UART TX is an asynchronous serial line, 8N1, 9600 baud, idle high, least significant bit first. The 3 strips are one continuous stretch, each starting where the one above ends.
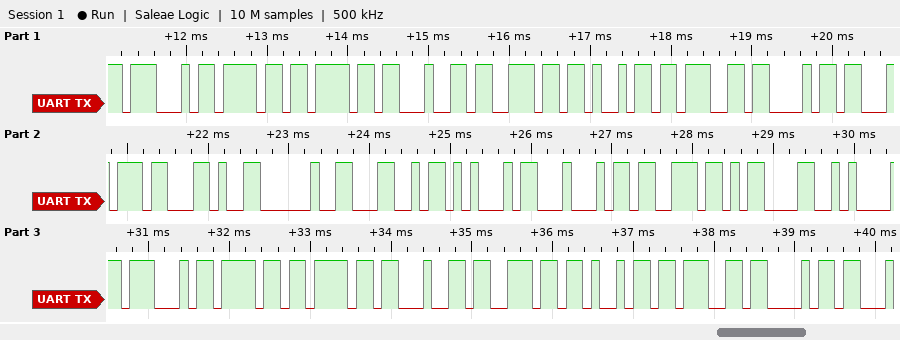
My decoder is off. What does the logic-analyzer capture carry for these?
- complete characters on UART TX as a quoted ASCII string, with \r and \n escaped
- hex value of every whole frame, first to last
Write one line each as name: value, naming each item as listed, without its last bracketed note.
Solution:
complete characters on UART TX as a quoted ASCII string, with \r and \n escaped: "Goodnight, LEDs\r\nGoodnigh"
hex value of every whole frame, first to last: 47 6F 6F 64 6E 69 67 68 74 2C 20 4C 45 44 73 0D 0A 47 6F 6F 64 6E 69 67 68
